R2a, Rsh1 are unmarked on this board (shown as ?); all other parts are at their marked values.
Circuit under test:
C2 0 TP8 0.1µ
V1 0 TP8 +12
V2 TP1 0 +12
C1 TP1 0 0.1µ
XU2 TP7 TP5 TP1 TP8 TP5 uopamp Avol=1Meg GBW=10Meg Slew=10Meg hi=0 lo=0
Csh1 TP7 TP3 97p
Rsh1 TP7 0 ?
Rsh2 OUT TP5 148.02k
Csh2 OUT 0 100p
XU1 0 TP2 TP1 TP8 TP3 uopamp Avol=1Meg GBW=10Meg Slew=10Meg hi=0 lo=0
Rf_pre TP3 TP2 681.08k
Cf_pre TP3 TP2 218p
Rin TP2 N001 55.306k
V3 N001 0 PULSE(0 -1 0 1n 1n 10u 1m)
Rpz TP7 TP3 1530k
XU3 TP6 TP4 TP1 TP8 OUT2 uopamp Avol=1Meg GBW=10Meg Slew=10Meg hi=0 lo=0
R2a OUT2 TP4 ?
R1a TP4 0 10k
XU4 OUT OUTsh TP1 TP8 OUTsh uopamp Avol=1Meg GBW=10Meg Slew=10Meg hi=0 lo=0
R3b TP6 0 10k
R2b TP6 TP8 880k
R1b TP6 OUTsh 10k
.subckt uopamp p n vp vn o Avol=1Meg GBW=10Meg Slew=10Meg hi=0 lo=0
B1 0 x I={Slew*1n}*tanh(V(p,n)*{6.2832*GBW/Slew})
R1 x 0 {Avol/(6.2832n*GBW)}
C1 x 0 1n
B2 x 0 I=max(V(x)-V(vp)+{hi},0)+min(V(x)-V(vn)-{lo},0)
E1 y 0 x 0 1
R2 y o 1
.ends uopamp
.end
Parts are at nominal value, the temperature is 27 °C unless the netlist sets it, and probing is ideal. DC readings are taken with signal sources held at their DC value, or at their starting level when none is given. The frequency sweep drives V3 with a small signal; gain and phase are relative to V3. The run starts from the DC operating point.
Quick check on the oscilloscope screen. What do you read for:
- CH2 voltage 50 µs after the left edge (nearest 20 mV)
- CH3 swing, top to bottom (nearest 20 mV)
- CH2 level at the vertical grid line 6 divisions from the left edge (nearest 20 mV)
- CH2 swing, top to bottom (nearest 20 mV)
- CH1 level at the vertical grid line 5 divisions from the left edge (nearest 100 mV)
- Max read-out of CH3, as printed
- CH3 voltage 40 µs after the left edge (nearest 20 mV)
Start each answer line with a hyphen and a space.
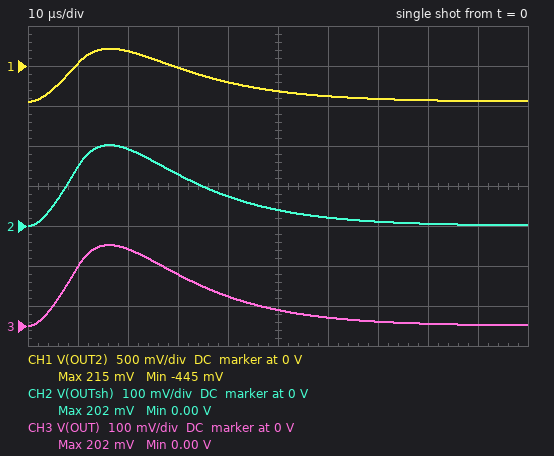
- 40 mV
- 200 mV
- 20 mV
- 200 mV
- -300 mV
- 202 mV
- 80 mV
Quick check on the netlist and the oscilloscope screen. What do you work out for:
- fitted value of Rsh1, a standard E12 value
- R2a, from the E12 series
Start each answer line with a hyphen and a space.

- 82 kΩ
- 56 kΩ
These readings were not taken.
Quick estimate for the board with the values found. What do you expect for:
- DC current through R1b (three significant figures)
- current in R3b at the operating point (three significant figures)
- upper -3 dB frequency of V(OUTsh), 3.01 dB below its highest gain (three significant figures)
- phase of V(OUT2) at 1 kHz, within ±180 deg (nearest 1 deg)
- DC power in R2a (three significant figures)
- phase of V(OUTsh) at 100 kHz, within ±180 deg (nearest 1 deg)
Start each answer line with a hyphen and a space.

- 6.78 µA
- 6.78 µA
- 8.93 kHz
- 172 deg
- 2.57 µW
- 16 deg
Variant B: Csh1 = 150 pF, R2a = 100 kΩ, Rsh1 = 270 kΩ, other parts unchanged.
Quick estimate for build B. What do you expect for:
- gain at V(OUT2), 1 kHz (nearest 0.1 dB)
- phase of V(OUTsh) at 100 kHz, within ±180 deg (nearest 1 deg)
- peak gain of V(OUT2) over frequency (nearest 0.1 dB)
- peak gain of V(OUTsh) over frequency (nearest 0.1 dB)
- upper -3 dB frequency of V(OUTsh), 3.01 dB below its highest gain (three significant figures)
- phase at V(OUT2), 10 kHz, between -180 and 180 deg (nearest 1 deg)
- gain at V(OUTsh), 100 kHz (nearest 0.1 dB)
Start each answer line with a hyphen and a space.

- 22.0 dB
- 7 deg
- 22.4 dB
- 7.7 dB
- 5.10 kHz
- 73 deg
- -37.0 dB
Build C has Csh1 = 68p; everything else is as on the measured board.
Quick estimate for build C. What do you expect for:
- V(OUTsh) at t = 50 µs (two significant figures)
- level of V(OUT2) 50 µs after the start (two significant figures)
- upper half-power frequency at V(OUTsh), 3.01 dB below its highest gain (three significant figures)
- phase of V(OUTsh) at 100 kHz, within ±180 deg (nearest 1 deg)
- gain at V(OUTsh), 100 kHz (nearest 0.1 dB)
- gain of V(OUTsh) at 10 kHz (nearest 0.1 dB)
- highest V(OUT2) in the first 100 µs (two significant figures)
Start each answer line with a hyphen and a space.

- 32 mV
- -340 mV
- 3.05 kHz
- 21 deg
- -37.4 dB
- -10.3 dB
- 85 mV
